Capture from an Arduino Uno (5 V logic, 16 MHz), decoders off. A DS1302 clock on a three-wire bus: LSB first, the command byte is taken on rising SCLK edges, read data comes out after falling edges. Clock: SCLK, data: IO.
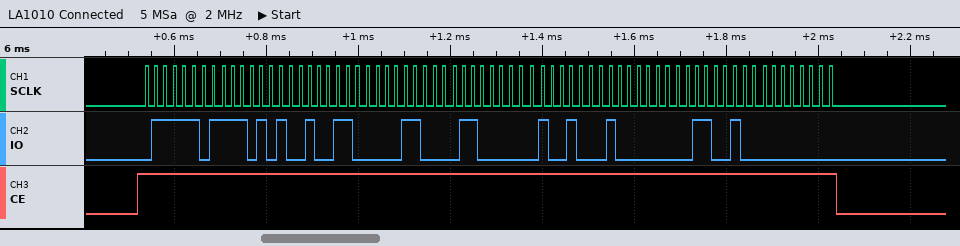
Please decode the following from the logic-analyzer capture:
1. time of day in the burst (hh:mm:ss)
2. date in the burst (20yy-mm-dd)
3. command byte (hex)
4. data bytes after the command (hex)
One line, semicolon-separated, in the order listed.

18:32:57; 2026-12-06; 0xBE; 57 32 18 06 12 01 26 00
